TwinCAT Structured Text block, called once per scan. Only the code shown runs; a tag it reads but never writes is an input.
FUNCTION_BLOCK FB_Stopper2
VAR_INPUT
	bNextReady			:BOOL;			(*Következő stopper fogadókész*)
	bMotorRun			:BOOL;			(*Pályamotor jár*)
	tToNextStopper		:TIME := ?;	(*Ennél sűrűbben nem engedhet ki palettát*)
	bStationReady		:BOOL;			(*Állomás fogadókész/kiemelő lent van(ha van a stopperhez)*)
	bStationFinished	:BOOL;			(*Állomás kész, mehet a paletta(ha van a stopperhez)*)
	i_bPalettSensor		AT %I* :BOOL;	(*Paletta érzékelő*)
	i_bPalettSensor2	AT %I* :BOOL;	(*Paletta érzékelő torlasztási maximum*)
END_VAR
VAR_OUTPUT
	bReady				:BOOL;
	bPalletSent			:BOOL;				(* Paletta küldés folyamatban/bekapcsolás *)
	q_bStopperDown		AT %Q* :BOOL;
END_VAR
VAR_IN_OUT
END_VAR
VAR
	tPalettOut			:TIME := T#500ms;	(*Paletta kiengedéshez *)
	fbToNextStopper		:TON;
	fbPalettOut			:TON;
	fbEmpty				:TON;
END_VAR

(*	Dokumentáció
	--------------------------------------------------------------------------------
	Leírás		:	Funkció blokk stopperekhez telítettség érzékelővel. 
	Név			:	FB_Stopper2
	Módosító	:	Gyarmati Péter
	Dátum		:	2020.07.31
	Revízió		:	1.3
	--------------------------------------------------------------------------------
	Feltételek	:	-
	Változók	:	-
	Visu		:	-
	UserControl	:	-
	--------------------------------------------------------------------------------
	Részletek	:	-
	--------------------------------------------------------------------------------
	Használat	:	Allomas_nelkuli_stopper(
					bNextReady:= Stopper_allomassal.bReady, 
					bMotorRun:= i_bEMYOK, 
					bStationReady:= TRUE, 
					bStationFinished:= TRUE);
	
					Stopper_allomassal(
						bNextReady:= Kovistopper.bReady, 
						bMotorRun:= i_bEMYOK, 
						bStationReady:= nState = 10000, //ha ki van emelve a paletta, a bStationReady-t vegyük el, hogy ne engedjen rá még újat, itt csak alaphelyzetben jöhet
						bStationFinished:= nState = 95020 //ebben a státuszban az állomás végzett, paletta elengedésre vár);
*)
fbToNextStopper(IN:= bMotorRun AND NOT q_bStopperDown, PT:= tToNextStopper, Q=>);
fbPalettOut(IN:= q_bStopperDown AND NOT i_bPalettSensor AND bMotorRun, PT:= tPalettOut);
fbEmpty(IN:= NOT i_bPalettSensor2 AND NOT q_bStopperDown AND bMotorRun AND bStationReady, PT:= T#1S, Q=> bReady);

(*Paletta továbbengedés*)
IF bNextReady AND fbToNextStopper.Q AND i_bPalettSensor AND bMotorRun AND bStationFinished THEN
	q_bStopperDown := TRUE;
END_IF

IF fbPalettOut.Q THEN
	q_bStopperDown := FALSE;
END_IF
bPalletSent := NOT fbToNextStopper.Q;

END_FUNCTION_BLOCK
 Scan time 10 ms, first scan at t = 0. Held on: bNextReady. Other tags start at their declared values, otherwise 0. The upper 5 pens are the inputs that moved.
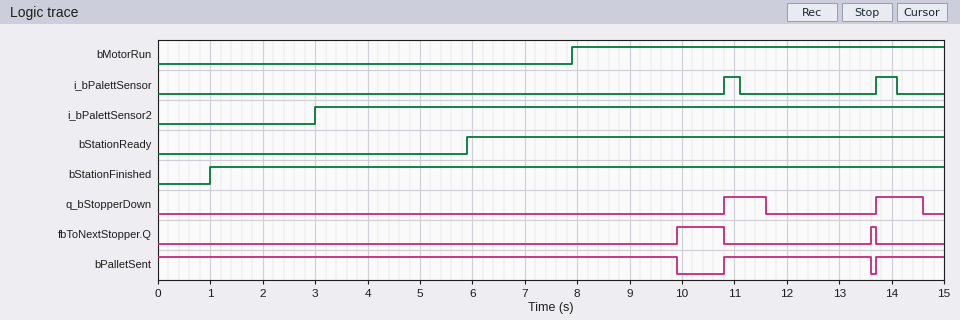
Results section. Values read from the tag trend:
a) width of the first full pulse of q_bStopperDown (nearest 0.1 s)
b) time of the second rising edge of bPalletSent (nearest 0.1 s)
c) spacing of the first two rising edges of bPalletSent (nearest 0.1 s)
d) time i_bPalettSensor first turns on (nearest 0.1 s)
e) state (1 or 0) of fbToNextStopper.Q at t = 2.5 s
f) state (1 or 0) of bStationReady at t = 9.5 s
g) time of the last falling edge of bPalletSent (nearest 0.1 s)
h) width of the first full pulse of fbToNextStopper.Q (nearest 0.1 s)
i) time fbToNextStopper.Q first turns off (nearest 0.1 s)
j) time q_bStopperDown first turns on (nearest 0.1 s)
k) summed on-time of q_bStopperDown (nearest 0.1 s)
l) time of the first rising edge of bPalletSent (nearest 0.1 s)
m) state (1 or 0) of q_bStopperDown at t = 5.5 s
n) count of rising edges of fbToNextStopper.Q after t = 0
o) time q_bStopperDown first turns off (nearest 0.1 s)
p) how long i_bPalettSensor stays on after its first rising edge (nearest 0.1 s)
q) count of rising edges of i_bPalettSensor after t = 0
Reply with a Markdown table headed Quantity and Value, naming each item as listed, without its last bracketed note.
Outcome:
| Quantity | Value |
|---|---|
| width of the first full pulse of q_bStopperDown | 0.8 s |
| time of the second rising edge of bPalletSent | 13.7 s |
| spacing of the first two rising edges of bPalletSent | 2.9 s |
| time i_bPalettSensor first turns on | 10.8 s |
| state (1 or 0) of fbToNextStopper.Q at t = 2.5 s | 0 |
| state (1 or 0) of bStationReady at t = 9.5 s | 1 |
| time of the last falling edge of bPalletSent | 13.6 s |
| width of the first full pulse of fbToNextStopper.Q | 0.9 s |
| time fbToNextStopper.Q first turns off | 10.8 s |
| time q_bStopperDown first turns on | 10.8 s |
| summed on-time of q_bStopperDown | 1.7 s |
| time of the first rising edge of bPalletSent | 10.8 s |
| state (1 or 0) of q_bStopperDown at t = 5.5 s | 0 |
| count of rising edges of fbToNextStopper.Q after t = 0 | 2 |
| time q_bStopperDown first turns off | 11.6 s |
| how long i_bPalettSensor stays on after its first rising edge | 0.3 s |
| count of rising edges of i_bPalettSensor after t = 0 | 2 |
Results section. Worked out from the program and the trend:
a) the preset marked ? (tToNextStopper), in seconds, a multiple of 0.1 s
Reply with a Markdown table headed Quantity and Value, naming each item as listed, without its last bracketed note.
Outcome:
| Quantity | Value |
|---|---|
| the preset marked ? (tToNextStopper), in seconds, a multiple of 0.1 s | 2.0 s |
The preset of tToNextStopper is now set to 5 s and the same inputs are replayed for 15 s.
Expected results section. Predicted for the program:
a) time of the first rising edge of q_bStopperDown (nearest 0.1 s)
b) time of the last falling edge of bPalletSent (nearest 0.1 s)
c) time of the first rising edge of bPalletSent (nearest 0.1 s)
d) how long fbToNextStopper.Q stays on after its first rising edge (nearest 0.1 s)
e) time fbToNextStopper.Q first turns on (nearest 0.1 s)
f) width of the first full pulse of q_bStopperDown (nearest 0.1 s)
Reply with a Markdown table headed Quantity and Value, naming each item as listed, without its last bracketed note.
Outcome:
| Quantity | Value |
|---|---|
| time of the first rising edge of q_bStopperDown | 13.7 s |
| time of the last falling edge of bPalletSent | 12.9 s |
| time of the first rising edge of bPalletSent | 13.7 s |
| how long fbToNextStopper.Q stays on after its first rising edge | 0.8 s |
| time fbToNextStopper.Q first turns on | 12.9 s |
| width of the first full pulse of q_bStopperDown | 0.9 s |
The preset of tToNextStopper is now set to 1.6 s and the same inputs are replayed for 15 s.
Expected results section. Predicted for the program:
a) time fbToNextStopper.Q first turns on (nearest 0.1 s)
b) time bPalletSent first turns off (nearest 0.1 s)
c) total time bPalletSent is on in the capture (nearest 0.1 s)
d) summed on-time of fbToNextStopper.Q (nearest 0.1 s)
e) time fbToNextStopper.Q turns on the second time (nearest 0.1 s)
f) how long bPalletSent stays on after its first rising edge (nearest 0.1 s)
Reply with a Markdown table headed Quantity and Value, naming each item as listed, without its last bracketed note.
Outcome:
| Quantity | Value |
|---|---|
| time fbToNextStopper.Q first turns on | 9.5 s |
| time bPalletSent first turns off | 9.5 s |
| total time bPalletSent is on in the capture | 13.2 s |
| summed on-time of fbToNextStopper.Q | 1.8 s |
| time fbToNextStopper.Q turns on the second time | 13.2 s |
| how long bPalletSent stays on after its first rising edge | 2.4 s |
